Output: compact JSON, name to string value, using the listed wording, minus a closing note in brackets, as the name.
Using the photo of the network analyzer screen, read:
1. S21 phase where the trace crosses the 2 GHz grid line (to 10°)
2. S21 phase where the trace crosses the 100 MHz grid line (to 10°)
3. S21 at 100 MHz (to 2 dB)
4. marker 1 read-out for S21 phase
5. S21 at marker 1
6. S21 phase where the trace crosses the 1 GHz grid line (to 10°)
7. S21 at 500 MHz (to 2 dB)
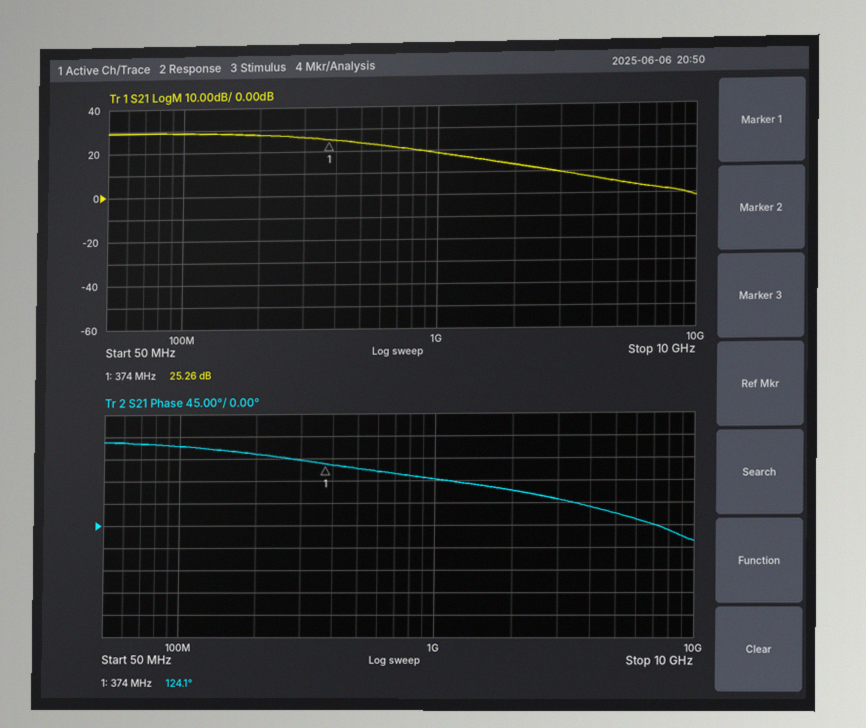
{"S21 phase where the trace crosses the 2 GHz grid line": "70°", "S21 phase where the trace crosses the 100 MHz grid line": "160°", "S21 at 100 MHz": "28 dB", "marker 1 read-out for S21 phase": "124.1°", "S21 at marker 1": "25.26 dB", "S21 phase where the trace crosses the 1 GHz grid line": "90°", "S21 at 500 MHz": "24 dB"}
